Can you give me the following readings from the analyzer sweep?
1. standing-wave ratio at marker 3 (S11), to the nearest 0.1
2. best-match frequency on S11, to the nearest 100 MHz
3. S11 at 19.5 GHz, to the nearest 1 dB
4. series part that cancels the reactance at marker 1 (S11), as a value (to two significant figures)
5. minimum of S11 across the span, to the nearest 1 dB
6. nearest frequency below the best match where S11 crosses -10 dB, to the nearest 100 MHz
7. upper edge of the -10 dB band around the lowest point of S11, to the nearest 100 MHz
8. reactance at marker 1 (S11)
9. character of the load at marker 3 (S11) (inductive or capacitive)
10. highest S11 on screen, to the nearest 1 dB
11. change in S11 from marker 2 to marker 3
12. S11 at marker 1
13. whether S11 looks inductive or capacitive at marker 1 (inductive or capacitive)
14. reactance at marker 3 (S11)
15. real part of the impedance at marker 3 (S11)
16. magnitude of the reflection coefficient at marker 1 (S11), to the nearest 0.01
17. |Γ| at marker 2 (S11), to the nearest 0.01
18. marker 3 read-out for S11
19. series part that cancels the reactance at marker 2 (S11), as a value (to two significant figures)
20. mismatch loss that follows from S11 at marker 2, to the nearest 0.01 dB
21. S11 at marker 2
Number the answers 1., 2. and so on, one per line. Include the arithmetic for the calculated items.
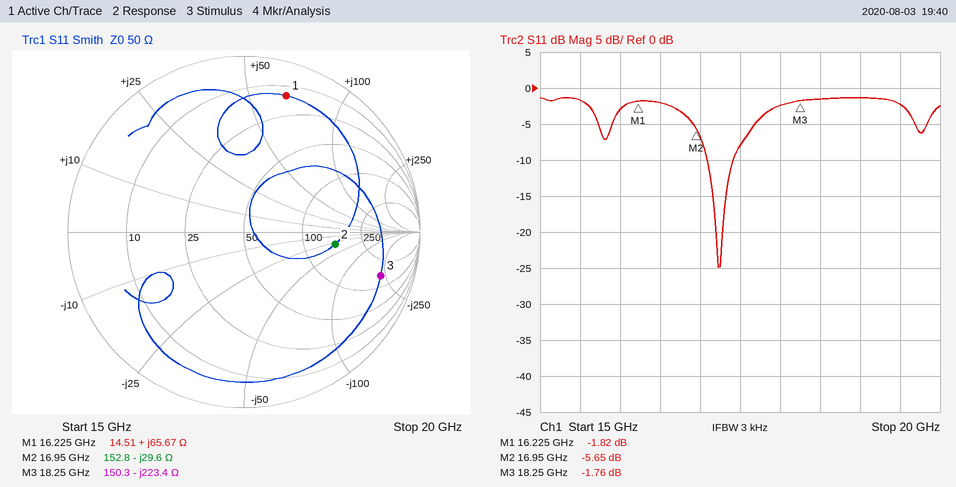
1. 9.9
2. 17.2 GHz
3. -2 dB
4. C = 1/(2π × 16.225 GHz × 65.67 Ω) ≈ 149 fF, so 150 fF to two significant figures
5. -25 dB
6. 17.1 GHz
7. 17.4 GHz
8. +65.67 Ω
9. capacitive
10. -1 dB
11. -1.76 − (-5.65) = 3.89 dB
12. -1.82 dB
13. inductive
14. -223.4 Ω
15. 150.3 Ω
16. 0.81
17. 0.52
18. -1.76 dB
19. L = 29.6 Ω/(2π × 16.95 GHz) ≈ 278 pH, so 280 pH to two significant figures
20. −10 log10(1 − 10^(-5.65/10)) ≈ 1.38 dB
21. -5.65 dB
